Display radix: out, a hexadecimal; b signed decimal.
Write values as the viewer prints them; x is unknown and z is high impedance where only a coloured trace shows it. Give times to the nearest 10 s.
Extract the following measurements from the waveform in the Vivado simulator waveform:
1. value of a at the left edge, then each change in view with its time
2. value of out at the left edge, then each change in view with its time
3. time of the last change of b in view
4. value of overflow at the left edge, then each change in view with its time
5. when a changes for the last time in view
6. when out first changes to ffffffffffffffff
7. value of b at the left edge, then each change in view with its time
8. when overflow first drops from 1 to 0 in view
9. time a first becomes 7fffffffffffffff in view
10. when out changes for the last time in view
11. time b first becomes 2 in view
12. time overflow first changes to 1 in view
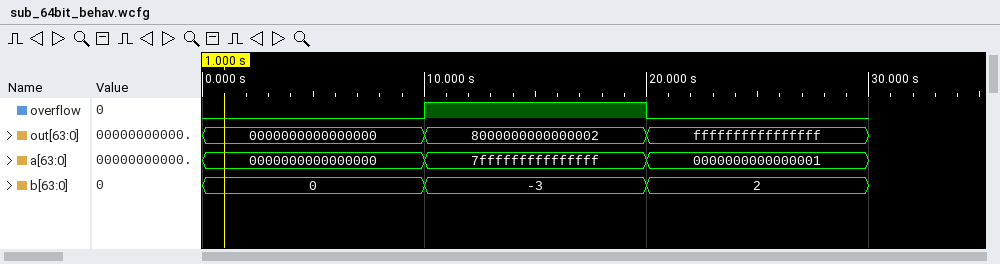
0000000000000000, 7fffffffffffffff at 10 s, 0000000000000001 at 20 s
0000000000000000, 8000000000000002 at 10 s, ffffffffffffffff at 20 s
20 s
0, 1 at 10 s, 0 at 20 s
20 s
20 s
0, -3 at 10 s, 2 at 20 s
20 s
10 s
20 s
20 s
10 s
